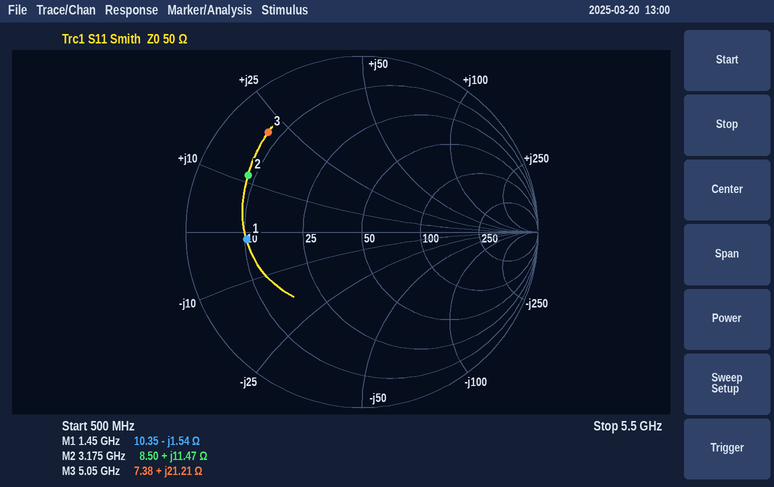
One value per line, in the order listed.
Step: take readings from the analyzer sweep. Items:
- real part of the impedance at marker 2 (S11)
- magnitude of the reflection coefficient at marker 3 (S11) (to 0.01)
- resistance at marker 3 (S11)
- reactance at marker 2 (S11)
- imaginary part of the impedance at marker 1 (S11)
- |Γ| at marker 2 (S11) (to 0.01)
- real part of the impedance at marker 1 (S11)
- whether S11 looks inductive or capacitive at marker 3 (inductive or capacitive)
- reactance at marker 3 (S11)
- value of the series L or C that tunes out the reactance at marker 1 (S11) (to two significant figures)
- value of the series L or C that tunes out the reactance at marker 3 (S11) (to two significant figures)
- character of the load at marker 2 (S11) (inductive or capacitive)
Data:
8.50 Ω
0.78
7.38 Ω
+11.47 Ω
-1.54 Ω
0.72
10.35 Ω
inductive
+21.21 Ω
170 pH
1.5 pF
inductive
